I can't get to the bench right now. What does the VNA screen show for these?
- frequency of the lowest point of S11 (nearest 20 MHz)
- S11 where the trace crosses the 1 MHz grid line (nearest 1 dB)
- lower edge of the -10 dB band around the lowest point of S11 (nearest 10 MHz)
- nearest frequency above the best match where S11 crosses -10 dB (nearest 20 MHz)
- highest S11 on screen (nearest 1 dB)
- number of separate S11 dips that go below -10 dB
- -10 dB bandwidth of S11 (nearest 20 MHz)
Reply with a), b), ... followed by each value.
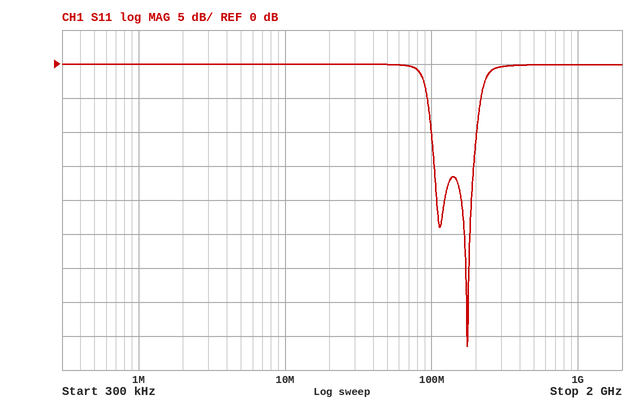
a) 180 MHz
b) 0 dB
c) 100 MHz
d) 200 MHz
e) 0 dB
f) 2
g) 100 MHz
